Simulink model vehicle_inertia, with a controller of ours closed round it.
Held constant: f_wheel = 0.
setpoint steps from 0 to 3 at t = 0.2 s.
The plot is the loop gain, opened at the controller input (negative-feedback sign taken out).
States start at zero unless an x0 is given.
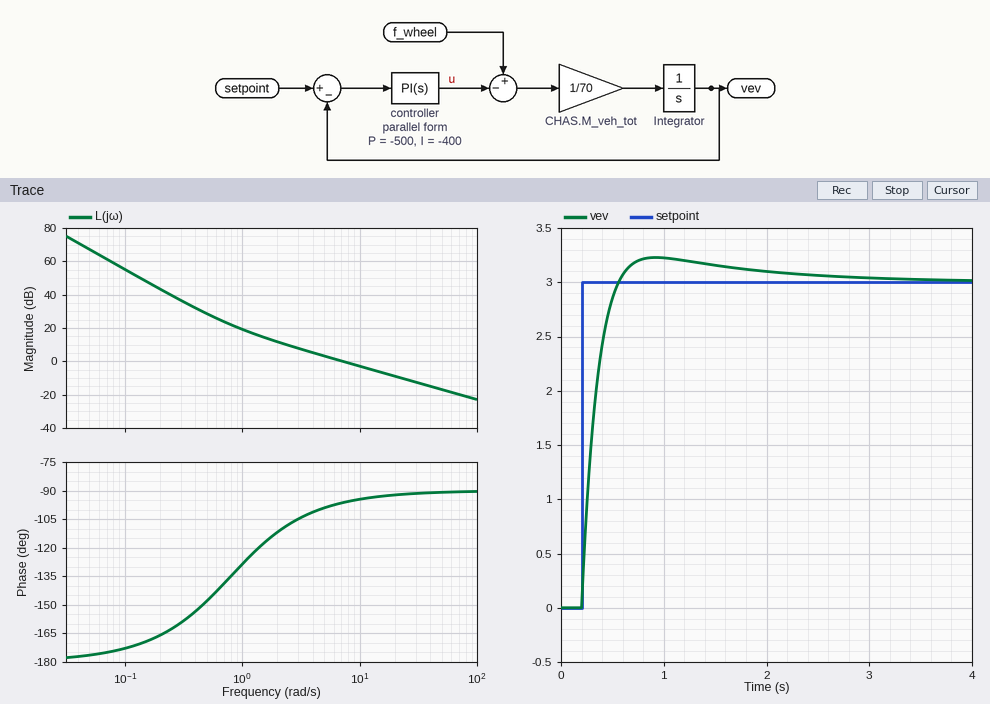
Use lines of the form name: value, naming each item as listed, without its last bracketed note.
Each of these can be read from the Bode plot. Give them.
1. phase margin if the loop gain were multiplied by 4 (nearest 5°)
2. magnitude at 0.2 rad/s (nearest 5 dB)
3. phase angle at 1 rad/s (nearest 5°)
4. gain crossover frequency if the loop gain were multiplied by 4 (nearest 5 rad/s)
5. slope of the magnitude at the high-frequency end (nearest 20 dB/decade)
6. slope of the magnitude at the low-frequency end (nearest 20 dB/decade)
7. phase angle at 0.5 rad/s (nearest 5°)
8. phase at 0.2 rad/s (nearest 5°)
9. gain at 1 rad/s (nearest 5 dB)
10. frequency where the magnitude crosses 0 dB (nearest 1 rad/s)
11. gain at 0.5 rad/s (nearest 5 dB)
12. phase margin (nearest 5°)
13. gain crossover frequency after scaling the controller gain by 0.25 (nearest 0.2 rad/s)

phase margin if the loop gain were multiplied by 4: 90°
magnitude at 0.2 rad/s: 45 dB
phase angle at 1 rad/s: -130°
gain crossover frequency if the loop gain were multiplied by 4: 30 rad/s
slope of the magnitude at the high-frequency end: -20 dB/decade
slope of the magnitude at the low-frequency end: -40 dB/decade
phase angle at 0.5 rad/s: -150°
phase at 0.2 rad/s: -165°
gain at 1 rad/s: 20 dB
frequency where the magnitude crosses 0 dB: 7 rad/s
gain at 0.5 rad/s: 30 dB
phase margin: 85°
gain crossover frequency after scaling the controller gain by 0.25: 2.0 rad/s
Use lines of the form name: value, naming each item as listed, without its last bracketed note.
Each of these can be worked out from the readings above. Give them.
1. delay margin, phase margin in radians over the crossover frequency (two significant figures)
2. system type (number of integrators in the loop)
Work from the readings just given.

delay margin, phase margin in radians over the crossover frequency: 0.21 s
system type: 2
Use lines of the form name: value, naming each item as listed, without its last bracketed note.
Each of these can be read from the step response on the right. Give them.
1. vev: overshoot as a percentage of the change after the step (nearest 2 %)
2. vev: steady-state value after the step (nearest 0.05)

vev: overshoot as a percentage of the change after the step: 8 %
vev: steady-state value after the step: 3.00
